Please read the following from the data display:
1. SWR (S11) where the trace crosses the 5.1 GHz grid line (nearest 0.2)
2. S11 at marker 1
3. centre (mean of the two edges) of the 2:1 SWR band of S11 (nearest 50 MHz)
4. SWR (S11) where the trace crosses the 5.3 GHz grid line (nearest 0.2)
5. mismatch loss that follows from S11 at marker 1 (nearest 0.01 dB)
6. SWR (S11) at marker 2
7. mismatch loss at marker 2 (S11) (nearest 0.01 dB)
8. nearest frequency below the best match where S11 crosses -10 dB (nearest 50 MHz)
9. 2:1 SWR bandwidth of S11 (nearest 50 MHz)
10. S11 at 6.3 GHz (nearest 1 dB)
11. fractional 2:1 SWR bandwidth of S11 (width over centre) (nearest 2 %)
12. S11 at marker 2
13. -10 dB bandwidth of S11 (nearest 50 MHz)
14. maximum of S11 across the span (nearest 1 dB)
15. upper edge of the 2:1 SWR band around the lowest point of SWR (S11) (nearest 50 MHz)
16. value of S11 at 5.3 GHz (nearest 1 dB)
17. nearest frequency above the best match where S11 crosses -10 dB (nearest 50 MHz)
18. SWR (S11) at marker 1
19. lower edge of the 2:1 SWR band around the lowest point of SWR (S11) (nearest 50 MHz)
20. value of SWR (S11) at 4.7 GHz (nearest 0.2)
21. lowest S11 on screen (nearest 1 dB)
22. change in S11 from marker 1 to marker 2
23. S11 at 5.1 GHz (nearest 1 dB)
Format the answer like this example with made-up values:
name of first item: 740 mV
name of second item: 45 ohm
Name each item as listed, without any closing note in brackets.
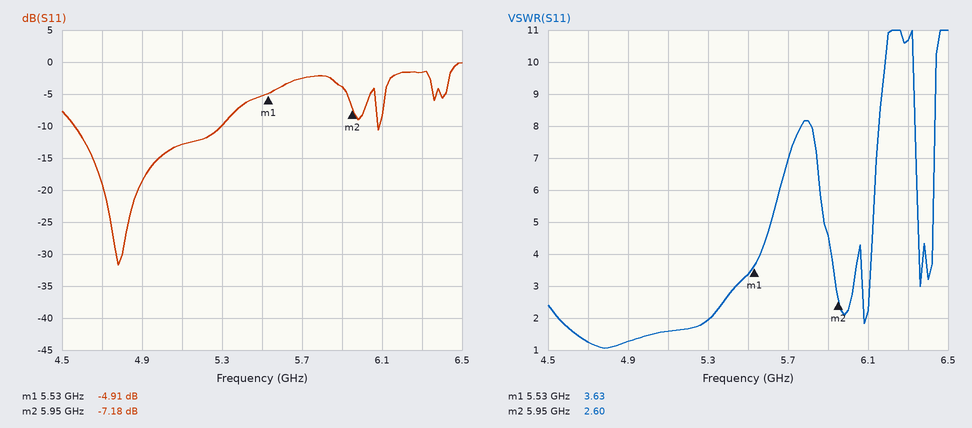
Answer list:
SWR (S11) where the trace crosses the 5.1 GHz grid line: 1.6
S11 at marker 1: -4.91 dB
centre (mean of the two edges) of the 2:1 SWR band of S11: 4.95 GHz
SWR (S11) where the trace crosses the 5.3 GHz grid line: 2.0
mismatch loss that follows from S11 at marker 1: 1.69 dB
SWR (S11) at marker 2: 2.60
mismatch loss at marker 2 (S11): 0.92 dB
nearest frequency below the best match where S11 crosses -10 dB: 4.55 GHz
2:1 SWR bandwidth of S11: 750 MHz
S11 at 6.3 GHz: -2 dB
fractional 2:1 SWR bandwidth of S11 (width over centre): 16 %
S11 at marker 2: -7.18 dB
-10 dB bandwidth of S11: 750 MHz
maximum of S11 across the span: 0 dB
upper edge of the 2:1 SWR band around the lowest point of SWR (S11): 5.30 GHz
value of S11 at 5.3 GHz: -10 dB
nearest frequency above the best match where S11 crosses -10 dB: 5.30 GHz
SWR (S11) at marker 1: 3.63
lower edge of the 2:1 SWR band around the lowest point of SWR (S11): 4.55 GHz
value of SWR (S11) at 4.7 GHz: 1.2
lowest S11 on screen: -32 dB
change in S11 from marker 1 to marker 2: -2.27 dB
S11 at 5.1 GHz: -13 dB
